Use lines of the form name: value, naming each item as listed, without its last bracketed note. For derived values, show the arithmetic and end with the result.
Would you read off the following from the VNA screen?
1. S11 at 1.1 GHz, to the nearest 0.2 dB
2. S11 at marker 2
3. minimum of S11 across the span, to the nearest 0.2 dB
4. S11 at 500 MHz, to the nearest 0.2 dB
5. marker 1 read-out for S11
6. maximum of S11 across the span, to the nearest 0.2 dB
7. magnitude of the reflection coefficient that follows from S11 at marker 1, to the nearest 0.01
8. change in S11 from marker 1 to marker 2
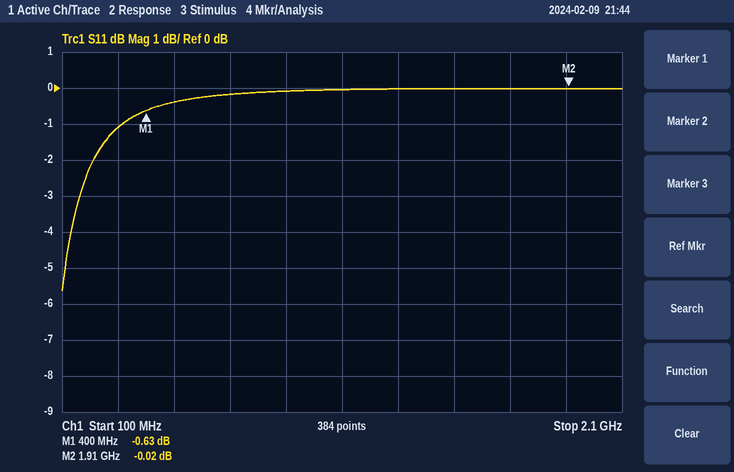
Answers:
S11 at 1.1 GHz, to the nearest 0.2 dB: 0.0 dB
S11 at marker 2: -0.02 dB
minimum of S11 across the span, to the nearest 0.2 dB: -5.6 dB
S11 at 500 MHz, to the nearest 0.2 dB: -0.4 dB
marker 1 read-out for S11: -0.63 dB
maximum of S11 across the span, to the nearest 0.2 dB: 0.0 dB
magnitude of the reflection coefficient that follows from S11 at marker 1, to the nearest 0.01: 10^(-0.63/20) ≈ 0.93
change in S11 from marker 1 to marker 2: -0.02 − (-0.63) = 0.61 dB
